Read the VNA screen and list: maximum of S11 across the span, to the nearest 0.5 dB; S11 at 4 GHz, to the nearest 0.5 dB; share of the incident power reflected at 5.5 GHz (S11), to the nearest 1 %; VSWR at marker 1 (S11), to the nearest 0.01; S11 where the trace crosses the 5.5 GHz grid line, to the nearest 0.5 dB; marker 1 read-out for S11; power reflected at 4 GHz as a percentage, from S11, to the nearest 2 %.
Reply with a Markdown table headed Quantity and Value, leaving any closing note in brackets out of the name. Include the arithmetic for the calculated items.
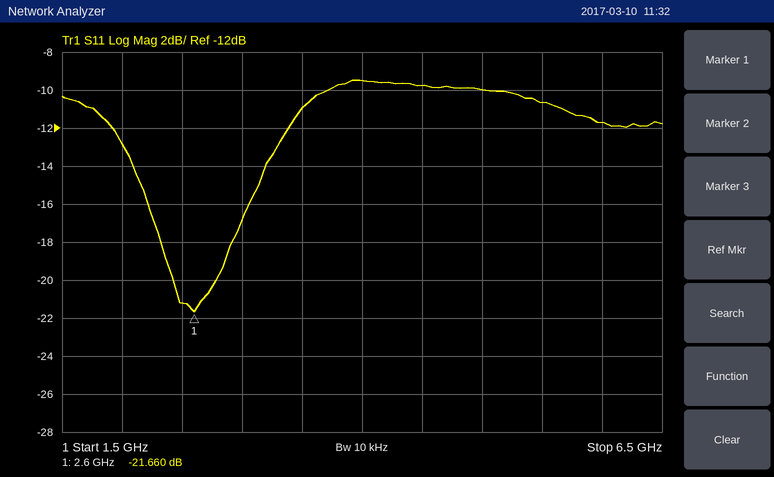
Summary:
| Quantity | Value |
|---|---|
| maximum of S11 across the span, to the nearest 0.5 dB | -9.5 dB |
| S11 at 4 GHz, to the nearest 0.5 dB | -9.5 dB |
| share of the incident power reflected at 5.5 GHz (S11), to the nearest 1 % | 10^(-10.5/10) ≈ 9 % |
| VSWR at marker 1 (S11), to the nearest 0.01 | (1 + 0.0826)/(1 − 0.0826) ≈ 1.18 |
| S11 where the trace crosses the 5.5 GHz grid line, to the nearest 0.5 dB | -10.5 dB |
| marker 1 read-out for S11 | -21.660 dB |
| power reflected at 4 GHz as a percentage, from S11, to the nearest 2 % | 10^(-9.5/10) ≈ 11.2 %, so 12 % to the nearest 2 % |
